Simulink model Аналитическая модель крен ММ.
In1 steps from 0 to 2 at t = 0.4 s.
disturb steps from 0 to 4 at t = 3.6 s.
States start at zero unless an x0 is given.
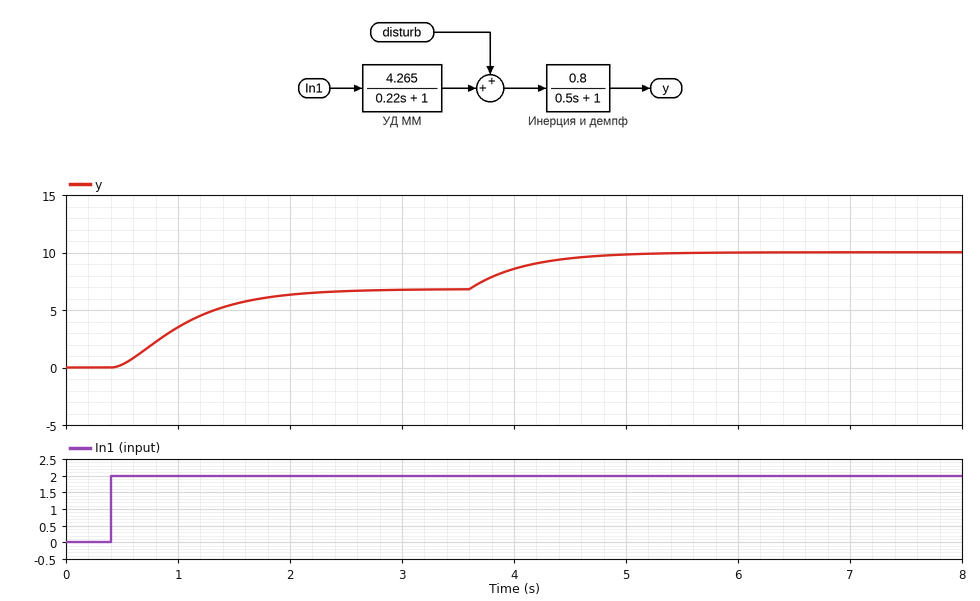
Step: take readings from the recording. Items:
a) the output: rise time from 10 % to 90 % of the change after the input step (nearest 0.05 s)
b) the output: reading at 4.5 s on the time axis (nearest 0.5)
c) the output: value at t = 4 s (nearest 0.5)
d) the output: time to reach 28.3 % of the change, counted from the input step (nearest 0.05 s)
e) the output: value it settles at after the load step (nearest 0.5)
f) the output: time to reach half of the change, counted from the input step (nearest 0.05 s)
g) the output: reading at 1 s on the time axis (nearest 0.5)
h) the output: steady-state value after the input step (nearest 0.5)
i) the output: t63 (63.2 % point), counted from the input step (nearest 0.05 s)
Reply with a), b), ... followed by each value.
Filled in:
a) 1.25 s
b) 9.5
c) 8.5
d) 0.35 s
e) 10.0
f) 0.60 s
g) 3.5
h) 7.0
i) 0.75 s
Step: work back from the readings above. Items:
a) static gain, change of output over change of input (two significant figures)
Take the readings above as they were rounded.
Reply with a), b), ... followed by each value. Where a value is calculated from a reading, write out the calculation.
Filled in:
a) (7 - 0) / (2 - 0) = 3.5
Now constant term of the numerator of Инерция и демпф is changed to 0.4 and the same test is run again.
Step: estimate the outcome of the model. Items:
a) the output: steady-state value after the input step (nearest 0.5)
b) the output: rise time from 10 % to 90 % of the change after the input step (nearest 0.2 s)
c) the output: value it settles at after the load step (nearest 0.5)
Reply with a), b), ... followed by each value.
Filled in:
a) 3.5
b) 1.2 s
c) 5.0
